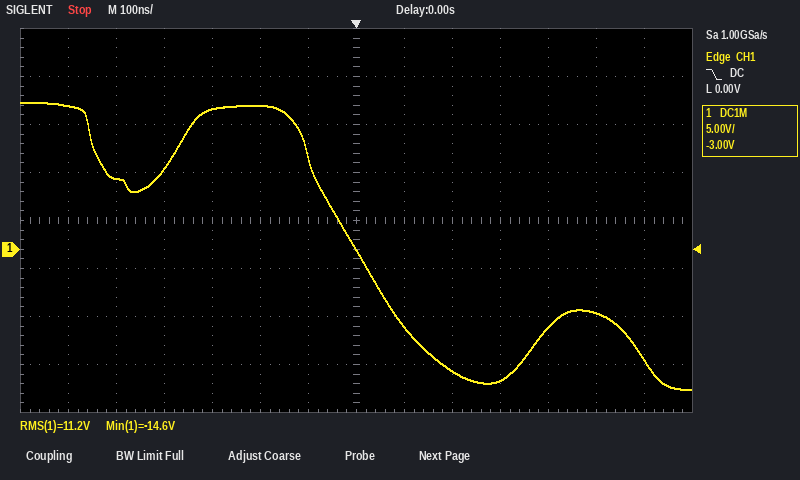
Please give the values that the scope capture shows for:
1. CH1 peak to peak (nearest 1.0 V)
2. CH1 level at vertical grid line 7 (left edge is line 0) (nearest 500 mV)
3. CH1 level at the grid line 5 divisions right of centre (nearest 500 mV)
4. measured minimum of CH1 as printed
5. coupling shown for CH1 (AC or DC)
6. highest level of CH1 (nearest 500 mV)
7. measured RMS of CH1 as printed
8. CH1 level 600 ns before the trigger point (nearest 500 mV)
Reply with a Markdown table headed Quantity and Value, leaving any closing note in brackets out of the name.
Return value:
| Quantity | Value |
|---|---|
| CH1 peak to peak | 30.0 V |
| CH1 level at vertical grid line 7 (left edge is line 0) | 0.0 V |
| CH1 level at the grid line 5 divisions right of centre | -6.5 V |
| measured minimum of CH1 as printed | -14.6 V |
| coupling shown for CH1 | DC |
| highest level of CH1 | 15.5 V |
| measured RMS of CH1 as printed | 11.2 V |
| CH1 level 600 ns before the trigger point | 15.0 V |
